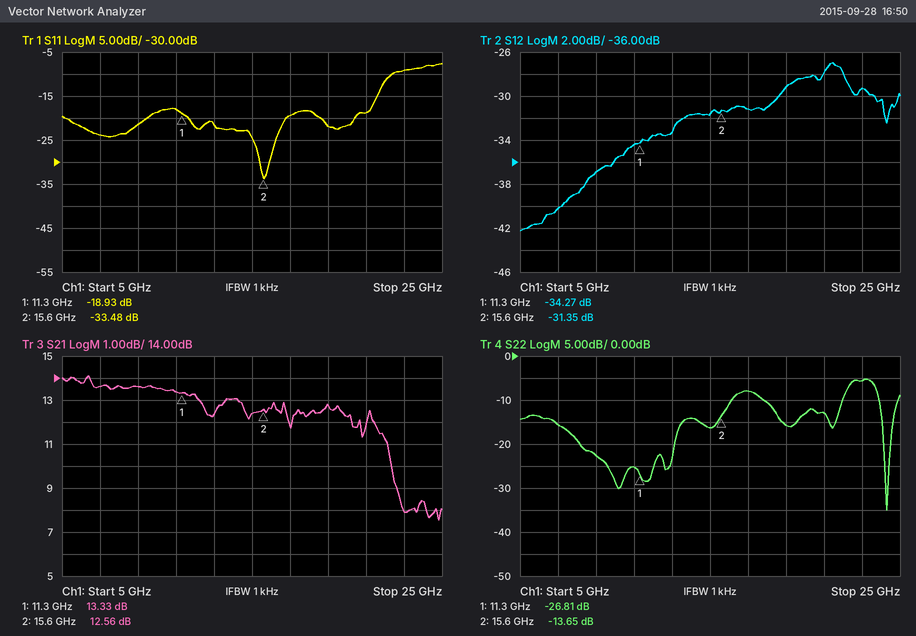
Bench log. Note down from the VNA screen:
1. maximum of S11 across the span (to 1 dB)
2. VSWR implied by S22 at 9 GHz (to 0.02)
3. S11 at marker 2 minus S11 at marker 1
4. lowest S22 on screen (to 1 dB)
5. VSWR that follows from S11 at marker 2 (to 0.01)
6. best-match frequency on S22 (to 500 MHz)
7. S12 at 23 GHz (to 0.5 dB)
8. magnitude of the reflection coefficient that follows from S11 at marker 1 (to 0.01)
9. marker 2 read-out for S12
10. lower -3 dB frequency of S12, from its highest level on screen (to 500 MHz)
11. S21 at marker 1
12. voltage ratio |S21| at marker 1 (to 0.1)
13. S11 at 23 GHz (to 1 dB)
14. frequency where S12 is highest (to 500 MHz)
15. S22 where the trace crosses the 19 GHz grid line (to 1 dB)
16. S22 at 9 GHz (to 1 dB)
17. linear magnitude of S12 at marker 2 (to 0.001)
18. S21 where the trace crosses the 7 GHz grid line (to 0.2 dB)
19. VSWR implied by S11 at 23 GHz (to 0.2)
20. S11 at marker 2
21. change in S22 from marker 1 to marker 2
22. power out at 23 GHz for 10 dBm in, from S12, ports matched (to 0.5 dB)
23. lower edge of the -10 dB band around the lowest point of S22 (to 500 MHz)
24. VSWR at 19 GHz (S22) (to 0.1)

-8 dB
1.16
-14.55 dB
-35 dB
1.04
24.5 GHz
-29.5 dB
0.11
-31.35 dB
18.5 GHz
13.33 dB
4.6
-9 dB
21.5 GHz
-16 dB
-23 dB
0.027
13.6 dB
2.0
-33.48 dB
13.16 dB
-19.5 dBm
24.0 GHz
1.4
